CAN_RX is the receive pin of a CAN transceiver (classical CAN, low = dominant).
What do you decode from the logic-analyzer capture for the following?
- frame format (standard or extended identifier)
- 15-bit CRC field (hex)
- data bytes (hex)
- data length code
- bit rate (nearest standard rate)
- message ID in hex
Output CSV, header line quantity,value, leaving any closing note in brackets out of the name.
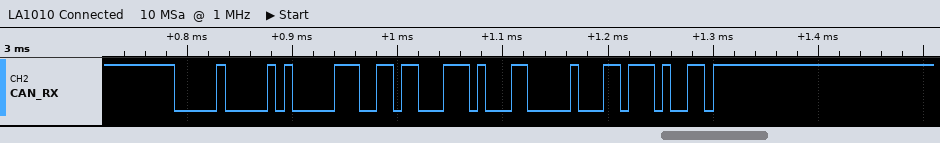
quantity,value
frame format,standard
15-bit CRC field,0x06E9
data bytes,36 3A 30
data length code,3
bit rate,125 kbit/s
message ID in hex,0x001
